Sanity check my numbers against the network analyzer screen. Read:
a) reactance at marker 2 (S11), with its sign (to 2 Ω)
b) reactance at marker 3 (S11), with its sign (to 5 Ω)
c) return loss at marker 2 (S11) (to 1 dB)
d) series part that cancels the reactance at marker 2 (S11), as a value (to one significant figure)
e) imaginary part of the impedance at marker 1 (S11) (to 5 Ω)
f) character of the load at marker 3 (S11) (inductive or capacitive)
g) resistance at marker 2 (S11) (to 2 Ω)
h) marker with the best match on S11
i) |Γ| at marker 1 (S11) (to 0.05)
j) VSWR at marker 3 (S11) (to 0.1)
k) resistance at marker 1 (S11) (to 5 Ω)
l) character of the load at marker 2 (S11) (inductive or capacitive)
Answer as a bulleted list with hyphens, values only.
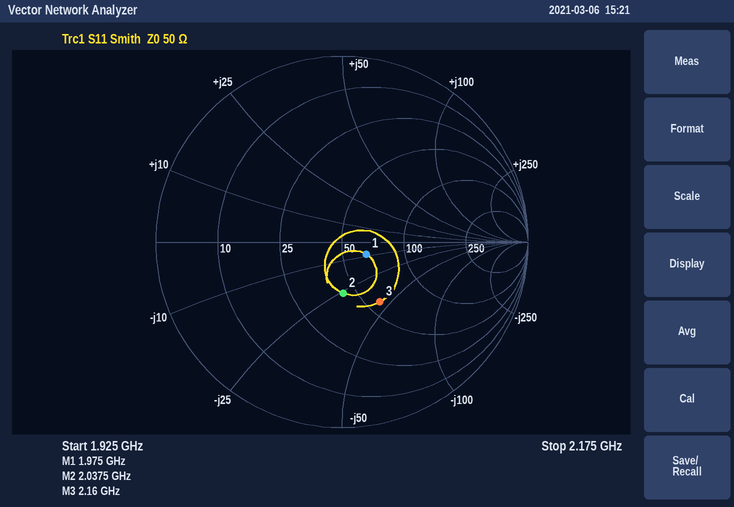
- -26 Ω
- -45 Ω
- 11 dB
- 2 nH
- -10 Ω
- capacitive
- 44 Ω
- marker 1
- 0.15
- 2.2
- 65 Ω
- capacitive
